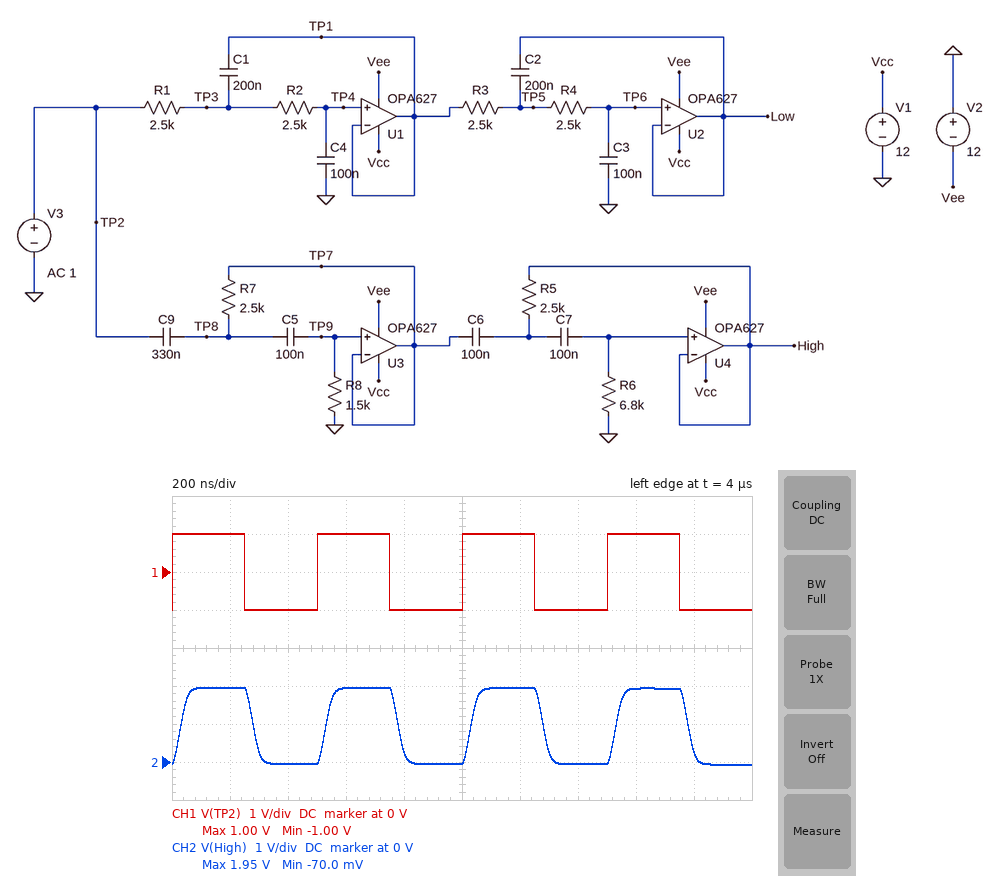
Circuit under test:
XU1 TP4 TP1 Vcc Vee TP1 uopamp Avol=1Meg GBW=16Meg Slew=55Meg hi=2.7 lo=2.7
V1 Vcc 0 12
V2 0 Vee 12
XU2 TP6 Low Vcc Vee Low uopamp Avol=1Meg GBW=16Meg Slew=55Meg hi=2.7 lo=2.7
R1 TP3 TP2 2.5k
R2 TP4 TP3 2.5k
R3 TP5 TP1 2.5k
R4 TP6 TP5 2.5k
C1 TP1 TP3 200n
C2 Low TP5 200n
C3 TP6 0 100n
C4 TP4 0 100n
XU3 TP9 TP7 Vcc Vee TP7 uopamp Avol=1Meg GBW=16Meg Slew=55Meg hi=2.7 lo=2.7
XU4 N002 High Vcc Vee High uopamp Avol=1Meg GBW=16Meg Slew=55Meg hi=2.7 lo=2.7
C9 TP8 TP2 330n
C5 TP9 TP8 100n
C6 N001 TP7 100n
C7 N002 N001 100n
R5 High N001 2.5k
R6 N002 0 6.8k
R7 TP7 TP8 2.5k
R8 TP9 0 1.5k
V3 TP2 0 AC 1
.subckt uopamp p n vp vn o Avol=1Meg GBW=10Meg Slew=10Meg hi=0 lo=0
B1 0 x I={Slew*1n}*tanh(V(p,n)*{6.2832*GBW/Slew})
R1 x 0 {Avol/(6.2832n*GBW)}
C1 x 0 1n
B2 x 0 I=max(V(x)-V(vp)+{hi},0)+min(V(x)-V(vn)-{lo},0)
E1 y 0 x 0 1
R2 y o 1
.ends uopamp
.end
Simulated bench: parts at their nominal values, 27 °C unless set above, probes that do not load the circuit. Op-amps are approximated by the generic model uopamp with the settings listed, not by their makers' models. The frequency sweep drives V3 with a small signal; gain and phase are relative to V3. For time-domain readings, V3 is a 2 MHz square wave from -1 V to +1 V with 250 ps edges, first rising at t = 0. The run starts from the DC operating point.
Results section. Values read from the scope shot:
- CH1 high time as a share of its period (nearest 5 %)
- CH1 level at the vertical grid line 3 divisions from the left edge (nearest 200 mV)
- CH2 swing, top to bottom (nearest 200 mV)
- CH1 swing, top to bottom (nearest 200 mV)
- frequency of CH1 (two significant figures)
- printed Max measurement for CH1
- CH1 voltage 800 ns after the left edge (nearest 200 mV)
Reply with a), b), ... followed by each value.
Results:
a) 50 %
b) 1.0 V
c) 2.0 V
d) 2.0 V
e) 2.0 MHz
f) 1.00 V
g) -1.0 V
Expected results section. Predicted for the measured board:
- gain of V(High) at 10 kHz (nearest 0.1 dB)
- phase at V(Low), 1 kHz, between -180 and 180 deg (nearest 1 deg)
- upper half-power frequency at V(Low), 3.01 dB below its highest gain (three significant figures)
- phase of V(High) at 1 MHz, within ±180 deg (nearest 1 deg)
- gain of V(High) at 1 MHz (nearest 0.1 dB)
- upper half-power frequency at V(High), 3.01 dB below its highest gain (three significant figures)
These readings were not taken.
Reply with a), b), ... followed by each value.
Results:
a) -0.1 dB
b) 77 deg
c) 361 Hz
d) -7 deg
e) 0 dB
f) 10.3 MHz
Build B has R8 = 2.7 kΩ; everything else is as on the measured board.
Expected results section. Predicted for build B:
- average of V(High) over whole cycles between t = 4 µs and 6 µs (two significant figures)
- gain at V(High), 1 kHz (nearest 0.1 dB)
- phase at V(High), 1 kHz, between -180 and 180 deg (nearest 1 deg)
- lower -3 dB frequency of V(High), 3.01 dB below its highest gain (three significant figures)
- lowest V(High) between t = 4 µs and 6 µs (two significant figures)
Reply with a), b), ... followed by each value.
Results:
a) 960 mV
b) -1.1 dB
c) 70 deg
d) 601 Hz
e) -46 mV
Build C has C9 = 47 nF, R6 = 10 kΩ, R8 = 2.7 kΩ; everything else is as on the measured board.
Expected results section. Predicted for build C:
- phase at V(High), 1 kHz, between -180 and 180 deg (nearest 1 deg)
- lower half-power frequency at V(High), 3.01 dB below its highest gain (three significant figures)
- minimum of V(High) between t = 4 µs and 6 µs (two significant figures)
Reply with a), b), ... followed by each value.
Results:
a) 103 deg
b) 1.39 kHz
c) -79 mV
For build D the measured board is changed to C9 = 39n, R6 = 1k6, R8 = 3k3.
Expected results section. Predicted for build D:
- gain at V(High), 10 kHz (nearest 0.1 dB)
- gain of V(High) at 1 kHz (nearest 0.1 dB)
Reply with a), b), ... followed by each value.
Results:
a) -0.2 dB
b) -10.9 dB
